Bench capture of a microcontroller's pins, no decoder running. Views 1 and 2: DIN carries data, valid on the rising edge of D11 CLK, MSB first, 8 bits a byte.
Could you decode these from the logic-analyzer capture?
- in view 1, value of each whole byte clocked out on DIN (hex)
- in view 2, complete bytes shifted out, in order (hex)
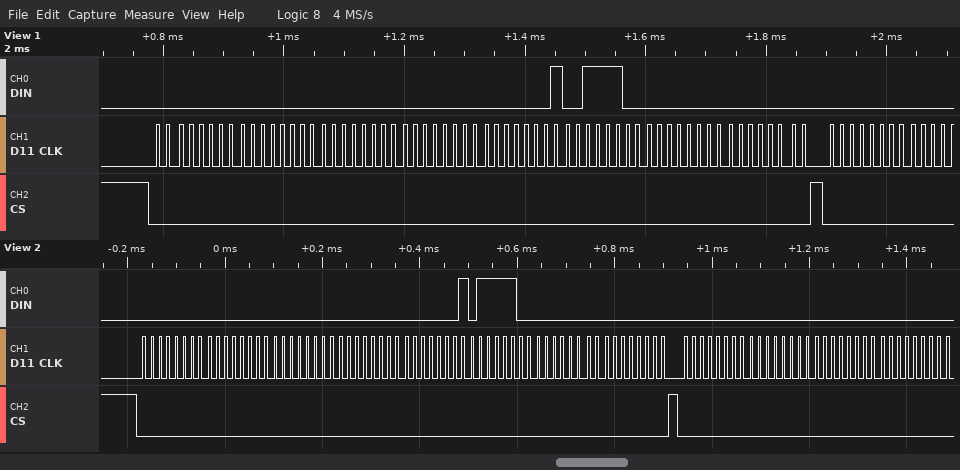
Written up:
00 00 00 00 01 3C 00 00 00
00 00 00 00 01 7C 00 00 00 00 00 00
